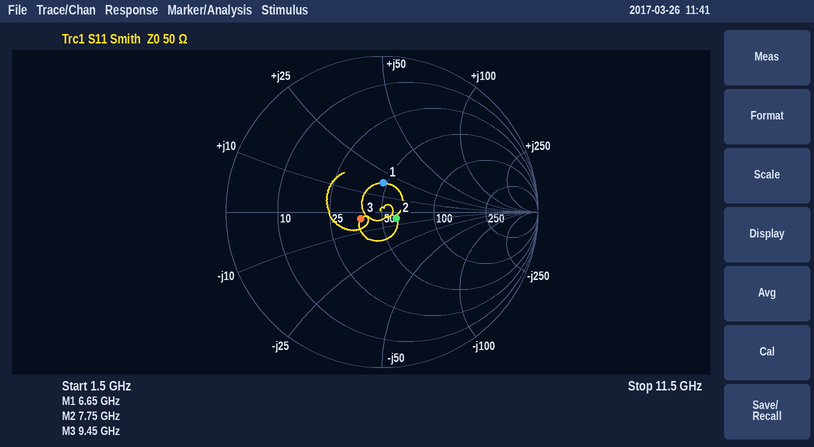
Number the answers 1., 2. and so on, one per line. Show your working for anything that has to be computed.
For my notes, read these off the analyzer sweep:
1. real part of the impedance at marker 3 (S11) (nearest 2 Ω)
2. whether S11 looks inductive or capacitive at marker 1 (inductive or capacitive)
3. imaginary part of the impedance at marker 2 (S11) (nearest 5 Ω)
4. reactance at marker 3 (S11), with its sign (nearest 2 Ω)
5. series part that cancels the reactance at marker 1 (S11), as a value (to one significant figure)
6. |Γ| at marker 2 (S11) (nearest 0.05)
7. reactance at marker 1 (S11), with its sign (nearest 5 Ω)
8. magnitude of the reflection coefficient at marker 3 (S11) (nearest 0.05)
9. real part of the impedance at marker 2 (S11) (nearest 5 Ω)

1. 38 Ω
2. inductive
3. -5 Ω
4. -4 Ω
5. C = 1/(2π × 6.65 GHz × 20 Ω) ≈ 1 pF
6. 0.10
7. +20 Ω
8. 0.15
9. 60 Ω
